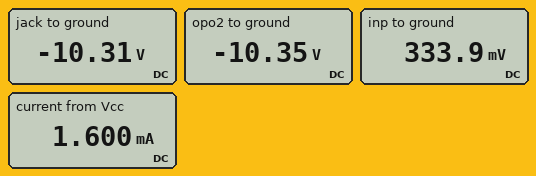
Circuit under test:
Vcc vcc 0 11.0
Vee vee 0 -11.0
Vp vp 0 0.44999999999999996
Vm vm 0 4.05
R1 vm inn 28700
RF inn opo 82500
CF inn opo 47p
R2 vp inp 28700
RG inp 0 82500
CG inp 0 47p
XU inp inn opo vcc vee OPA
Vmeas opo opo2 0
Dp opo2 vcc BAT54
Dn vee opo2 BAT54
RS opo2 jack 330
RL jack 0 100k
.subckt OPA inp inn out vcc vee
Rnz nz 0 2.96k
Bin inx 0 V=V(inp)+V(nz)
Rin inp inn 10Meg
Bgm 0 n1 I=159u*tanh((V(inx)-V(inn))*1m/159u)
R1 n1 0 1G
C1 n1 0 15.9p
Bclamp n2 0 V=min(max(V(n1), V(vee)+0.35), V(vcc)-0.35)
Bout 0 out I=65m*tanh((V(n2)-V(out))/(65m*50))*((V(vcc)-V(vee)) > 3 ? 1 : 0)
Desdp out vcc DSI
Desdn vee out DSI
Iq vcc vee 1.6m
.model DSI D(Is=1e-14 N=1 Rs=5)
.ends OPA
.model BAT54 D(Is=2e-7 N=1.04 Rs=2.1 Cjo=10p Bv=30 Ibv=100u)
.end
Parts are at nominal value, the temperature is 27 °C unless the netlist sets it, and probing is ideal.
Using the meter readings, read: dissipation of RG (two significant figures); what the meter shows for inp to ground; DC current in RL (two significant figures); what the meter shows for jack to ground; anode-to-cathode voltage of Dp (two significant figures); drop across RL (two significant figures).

1.4 µW
333.9 mV
100 µA
-10.31 V
-21 V
10 V
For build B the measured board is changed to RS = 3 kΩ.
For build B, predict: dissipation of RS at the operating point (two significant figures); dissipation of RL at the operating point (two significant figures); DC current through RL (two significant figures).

30 µW
1.0 mW
100 µA
